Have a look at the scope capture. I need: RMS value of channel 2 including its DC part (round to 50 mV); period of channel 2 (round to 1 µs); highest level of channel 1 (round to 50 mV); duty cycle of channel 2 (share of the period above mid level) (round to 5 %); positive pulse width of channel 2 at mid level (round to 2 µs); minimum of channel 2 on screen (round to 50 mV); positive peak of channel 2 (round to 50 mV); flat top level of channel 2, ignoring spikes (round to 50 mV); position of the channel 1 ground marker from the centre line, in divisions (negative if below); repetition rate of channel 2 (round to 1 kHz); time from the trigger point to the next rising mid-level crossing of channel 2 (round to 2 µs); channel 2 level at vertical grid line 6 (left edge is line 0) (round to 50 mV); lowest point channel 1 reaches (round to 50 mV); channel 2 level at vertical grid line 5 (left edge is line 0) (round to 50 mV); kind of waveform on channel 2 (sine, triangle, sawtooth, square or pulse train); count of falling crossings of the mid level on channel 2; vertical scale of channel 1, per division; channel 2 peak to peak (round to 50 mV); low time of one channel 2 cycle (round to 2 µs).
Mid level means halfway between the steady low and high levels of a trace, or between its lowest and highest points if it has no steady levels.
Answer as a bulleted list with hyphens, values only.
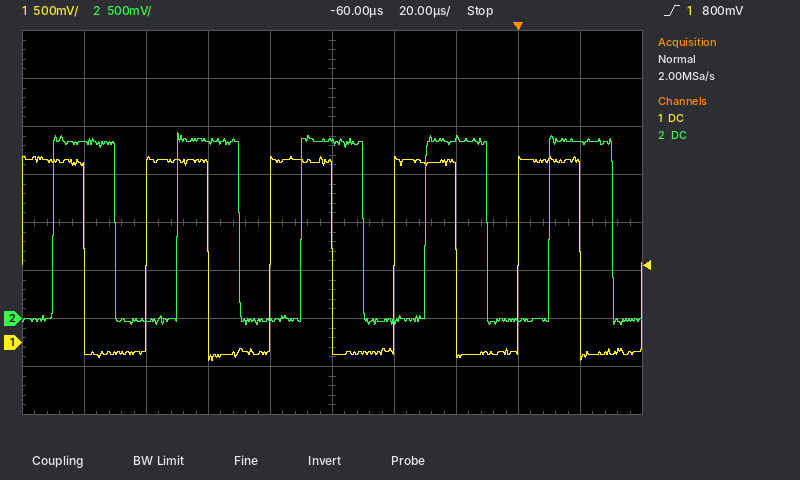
- 1.30 V
- 40 µs
- 1.95 V
- 50 %
- 20 µs
- -50 mV
- 1.95 V
- 1.85 V
- -2.5 div
- 25 kHz
- 10 µs
- -50 mV
- -200 mV
- 1.85 V
- square
- 5
- 500 mV
- 2.00 V
- 20 µs
